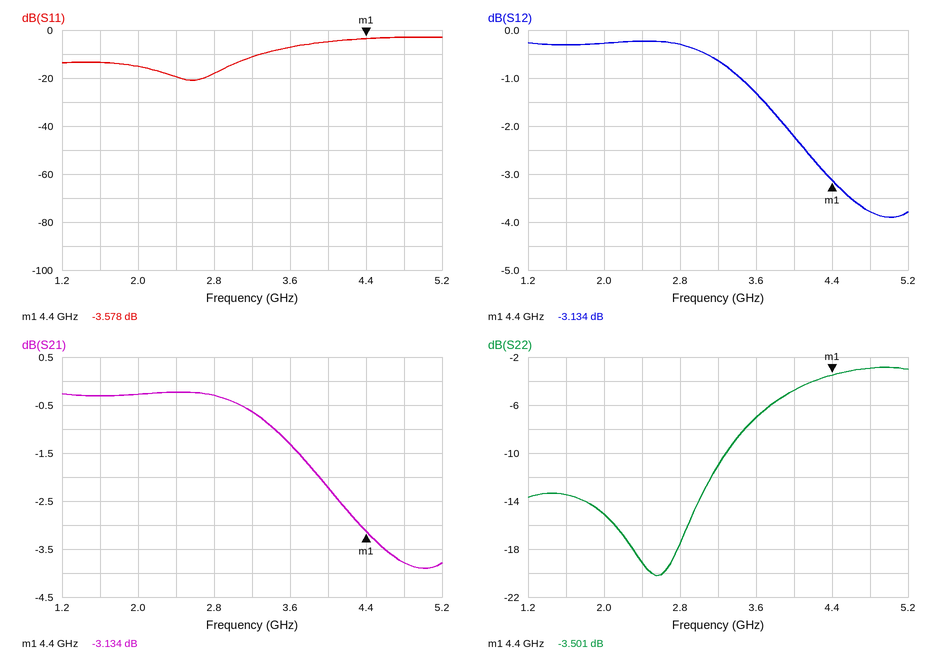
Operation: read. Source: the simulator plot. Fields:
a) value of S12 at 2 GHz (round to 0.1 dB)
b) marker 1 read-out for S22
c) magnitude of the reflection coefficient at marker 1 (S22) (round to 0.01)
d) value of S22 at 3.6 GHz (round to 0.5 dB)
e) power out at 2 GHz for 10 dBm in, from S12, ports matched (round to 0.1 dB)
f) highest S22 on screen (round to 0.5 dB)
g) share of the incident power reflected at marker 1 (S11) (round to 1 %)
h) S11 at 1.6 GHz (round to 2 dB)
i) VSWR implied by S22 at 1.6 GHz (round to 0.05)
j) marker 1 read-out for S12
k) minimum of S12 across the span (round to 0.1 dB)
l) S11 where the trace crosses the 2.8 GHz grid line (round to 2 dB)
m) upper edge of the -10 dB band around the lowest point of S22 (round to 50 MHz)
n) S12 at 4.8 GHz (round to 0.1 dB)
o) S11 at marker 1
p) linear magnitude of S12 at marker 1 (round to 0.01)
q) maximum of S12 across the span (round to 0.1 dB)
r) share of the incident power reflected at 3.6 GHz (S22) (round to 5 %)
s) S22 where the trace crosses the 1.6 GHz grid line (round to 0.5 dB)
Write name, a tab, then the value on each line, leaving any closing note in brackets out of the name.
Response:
value of S12 at 2 GHz	-0.3 dB
marker 1 read-out for S22	-3.501 dB
magnitude of the reflection coefficient at marker 1 (S22)	0.67
value of S22 at 3.6 GHz	-7.0 dB
power out at 2 GHz for 10 dBm in, from S12, ports matched	9.7 dBm
highest S22 on screen	-3.0 dB
share of the incident power reflected at marker 1 (S11)	44 %
S11 at 1.6 GHz	-14 dB
VSWR implied by S22 at 1.6 GHz	1.55
marker 1 read-out for S12	-3.134 dB
minimum of S12 across the span	-3.9 dB
S11 where the trace crosses the 2.8 GHz grid line	-18 dB
upper edge of the -10 dB band around the lowest point of S22	3.30 GHz
S12 at 4.8 GHz	-3.8 dB
S11 at marker 1	-3.578 dB
linear magnitude of S12 at marker 1	0.70
maximum of S12 across the span	-0.2 dB
share of the incident power reflected at 3.6 GHz (S22)	20 %
S22 where the trace crosses the 1.6 GHz grid line	-13.5 dB
